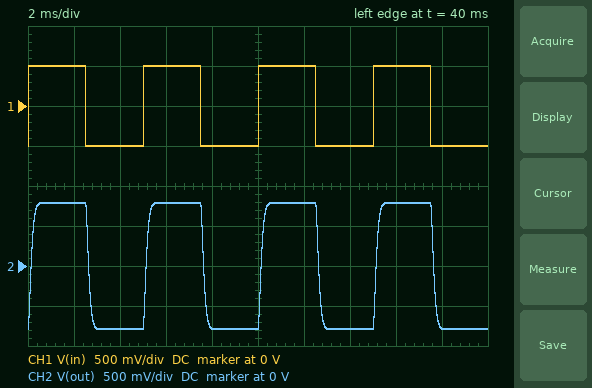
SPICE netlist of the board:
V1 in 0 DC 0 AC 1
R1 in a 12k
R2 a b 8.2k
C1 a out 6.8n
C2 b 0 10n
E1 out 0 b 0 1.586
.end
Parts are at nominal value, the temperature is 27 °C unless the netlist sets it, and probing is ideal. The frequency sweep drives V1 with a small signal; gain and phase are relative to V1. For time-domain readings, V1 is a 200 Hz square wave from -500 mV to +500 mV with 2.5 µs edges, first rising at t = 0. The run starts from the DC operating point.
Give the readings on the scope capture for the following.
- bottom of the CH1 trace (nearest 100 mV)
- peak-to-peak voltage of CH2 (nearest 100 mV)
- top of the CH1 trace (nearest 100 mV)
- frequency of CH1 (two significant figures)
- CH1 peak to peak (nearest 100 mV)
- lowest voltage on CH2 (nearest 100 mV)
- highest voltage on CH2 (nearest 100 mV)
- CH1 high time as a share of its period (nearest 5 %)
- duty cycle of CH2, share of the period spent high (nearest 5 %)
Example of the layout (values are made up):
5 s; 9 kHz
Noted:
-500 mV; 1.6 V; 500 mV; 200 Hz; 1.0 V; -800 mV; 800 mV; 50 %; 50 %
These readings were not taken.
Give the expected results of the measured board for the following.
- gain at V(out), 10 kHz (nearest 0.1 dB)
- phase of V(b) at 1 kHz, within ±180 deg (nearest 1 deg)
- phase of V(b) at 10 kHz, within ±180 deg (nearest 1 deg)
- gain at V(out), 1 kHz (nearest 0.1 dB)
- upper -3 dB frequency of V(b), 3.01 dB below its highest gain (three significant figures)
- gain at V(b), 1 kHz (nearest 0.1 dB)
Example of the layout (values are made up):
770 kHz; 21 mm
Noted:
-24.7 dB; -53 deg; -159 deg; 2.3 dB; 1.36 kHz; -1.7 dB
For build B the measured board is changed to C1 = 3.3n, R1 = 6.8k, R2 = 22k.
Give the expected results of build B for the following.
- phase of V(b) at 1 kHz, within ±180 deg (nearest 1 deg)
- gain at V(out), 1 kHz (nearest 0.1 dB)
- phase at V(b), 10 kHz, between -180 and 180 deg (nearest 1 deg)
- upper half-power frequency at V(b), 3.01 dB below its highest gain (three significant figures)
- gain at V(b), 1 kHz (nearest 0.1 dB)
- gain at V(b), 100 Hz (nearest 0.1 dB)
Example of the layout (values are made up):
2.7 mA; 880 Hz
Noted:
-65 deg; -1.6 dB; -137 deg; 619 Hz; -5.6 dB; -0.1 dB
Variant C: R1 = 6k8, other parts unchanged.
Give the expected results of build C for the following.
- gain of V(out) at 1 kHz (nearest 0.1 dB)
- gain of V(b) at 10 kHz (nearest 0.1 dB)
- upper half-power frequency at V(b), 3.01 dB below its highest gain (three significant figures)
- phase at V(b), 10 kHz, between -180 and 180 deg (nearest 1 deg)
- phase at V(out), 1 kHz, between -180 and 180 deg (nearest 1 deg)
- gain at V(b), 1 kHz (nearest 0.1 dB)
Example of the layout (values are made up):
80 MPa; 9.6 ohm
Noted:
2.8 dB; -24.1 dB; 1.67 kHz; -151 deg; -42 deg; -1.2 dB
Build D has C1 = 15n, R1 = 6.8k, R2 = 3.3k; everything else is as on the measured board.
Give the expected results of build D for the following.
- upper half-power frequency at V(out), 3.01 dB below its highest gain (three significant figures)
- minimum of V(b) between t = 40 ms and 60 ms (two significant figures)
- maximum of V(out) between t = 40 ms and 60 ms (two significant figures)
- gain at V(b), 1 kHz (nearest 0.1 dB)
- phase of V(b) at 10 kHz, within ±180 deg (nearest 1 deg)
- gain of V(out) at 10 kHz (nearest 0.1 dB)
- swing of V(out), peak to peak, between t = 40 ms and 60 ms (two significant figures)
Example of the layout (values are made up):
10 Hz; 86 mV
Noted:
3.26 kHz; -810 mV; 1.3 V; 0.9 dB; -168 deg; -18.0 dB; 2.6 V
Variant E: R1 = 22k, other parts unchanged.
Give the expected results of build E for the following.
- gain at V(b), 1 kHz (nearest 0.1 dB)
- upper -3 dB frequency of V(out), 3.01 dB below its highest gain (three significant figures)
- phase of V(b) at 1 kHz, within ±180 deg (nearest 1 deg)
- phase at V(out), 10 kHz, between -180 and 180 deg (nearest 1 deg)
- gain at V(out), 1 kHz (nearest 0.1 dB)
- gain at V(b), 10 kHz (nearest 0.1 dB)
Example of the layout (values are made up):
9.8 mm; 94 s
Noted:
-3.2 dB; 969 Hz; -69 deg; -164 deg; 0.8 dB; -33.9 dB
